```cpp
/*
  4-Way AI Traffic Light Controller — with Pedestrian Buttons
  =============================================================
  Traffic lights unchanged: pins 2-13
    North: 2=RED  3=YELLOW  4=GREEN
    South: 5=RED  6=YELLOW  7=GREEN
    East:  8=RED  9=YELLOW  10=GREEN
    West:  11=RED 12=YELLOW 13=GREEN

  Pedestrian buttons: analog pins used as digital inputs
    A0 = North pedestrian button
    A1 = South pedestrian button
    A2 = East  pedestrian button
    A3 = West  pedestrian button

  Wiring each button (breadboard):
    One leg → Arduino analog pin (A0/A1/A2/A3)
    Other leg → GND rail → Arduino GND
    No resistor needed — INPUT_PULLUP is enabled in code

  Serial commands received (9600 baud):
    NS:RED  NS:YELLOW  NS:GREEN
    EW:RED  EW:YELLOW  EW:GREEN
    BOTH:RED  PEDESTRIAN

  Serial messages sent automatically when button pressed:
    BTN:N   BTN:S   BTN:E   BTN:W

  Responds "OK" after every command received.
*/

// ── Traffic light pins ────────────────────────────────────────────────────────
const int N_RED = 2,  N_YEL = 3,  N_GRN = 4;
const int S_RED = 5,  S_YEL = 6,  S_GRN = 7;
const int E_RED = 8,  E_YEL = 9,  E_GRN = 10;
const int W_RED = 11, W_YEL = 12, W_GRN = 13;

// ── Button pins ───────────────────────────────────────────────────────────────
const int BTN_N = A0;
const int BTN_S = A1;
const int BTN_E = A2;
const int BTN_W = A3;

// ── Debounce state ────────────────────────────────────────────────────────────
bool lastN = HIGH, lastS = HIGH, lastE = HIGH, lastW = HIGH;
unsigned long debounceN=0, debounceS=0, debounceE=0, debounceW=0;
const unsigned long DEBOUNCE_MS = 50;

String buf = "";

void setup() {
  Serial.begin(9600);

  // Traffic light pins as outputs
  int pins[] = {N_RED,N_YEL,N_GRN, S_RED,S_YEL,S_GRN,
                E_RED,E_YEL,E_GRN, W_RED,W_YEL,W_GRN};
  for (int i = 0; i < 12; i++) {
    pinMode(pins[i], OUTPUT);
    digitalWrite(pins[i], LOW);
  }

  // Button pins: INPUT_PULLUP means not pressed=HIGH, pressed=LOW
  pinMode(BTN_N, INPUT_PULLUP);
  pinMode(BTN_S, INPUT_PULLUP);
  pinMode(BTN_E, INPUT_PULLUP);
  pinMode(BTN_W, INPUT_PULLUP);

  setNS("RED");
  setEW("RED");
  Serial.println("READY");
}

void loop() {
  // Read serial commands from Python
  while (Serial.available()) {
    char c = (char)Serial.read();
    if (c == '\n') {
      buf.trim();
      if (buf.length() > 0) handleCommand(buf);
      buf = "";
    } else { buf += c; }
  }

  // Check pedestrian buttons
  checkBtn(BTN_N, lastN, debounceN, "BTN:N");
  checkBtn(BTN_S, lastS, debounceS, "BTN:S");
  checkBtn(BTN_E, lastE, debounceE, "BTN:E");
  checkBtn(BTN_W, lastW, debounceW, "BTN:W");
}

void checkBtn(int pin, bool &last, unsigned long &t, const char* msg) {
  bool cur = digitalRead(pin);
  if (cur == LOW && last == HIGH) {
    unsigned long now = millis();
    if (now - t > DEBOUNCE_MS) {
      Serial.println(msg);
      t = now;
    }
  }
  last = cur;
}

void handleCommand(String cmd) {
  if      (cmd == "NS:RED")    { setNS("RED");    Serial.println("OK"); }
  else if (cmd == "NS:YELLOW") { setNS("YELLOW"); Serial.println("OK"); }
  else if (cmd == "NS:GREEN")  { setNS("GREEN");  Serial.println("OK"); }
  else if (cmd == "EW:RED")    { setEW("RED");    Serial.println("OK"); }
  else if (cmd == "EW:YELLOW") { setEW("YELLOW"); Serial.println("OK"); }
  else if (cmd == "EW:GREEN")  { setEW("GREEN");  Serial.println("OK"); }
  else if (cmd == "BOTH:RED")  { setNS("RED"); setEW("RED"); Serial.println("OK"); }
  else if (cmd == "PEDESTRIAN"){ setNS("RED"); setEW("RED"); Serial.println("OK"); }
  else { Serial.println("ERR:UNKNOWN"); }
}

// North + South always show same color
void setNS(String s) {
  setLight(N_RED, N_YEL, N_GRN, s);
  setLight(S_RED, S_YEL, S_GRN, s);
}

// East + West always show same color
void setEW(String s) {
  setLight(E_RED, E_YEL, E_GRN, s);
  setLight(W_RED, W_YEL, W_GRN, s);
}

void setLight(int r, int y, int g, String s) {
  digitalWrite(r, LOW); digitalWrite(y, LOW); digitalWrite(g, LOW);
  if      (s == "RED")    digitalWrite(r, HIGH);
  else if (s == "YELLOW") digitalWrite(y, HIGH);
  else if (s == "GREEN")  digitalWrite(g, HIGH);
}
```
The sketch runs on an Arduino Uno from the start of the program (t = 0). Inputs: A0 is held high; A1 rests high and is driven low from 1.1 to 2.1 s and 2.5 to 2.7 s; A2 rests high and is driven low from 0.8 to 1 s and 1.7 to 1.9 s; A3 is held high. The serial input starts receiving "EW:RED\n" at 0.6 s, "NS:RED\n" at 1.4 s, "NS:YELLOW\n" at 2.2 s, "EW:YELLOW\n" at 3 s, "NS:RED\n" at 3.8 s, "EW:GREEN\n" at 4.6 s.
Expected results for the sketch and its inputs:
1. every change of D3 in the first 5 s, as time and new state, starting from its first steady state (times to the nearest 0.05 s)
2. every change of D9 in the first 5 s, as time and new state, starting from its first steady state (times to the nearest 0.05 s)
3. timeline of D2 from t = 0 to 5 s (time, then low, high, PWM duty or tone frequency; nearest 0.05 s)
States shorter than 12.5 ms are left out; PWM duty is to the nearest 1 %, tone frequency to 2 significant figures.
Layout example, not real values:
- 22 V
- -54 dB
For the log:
- 0 s low; 2.2 s high; 3.8 s low
- 0 s low; 3 s high; 4.6 s low
- 0 s high; 2.2 s low; 3.8 s high
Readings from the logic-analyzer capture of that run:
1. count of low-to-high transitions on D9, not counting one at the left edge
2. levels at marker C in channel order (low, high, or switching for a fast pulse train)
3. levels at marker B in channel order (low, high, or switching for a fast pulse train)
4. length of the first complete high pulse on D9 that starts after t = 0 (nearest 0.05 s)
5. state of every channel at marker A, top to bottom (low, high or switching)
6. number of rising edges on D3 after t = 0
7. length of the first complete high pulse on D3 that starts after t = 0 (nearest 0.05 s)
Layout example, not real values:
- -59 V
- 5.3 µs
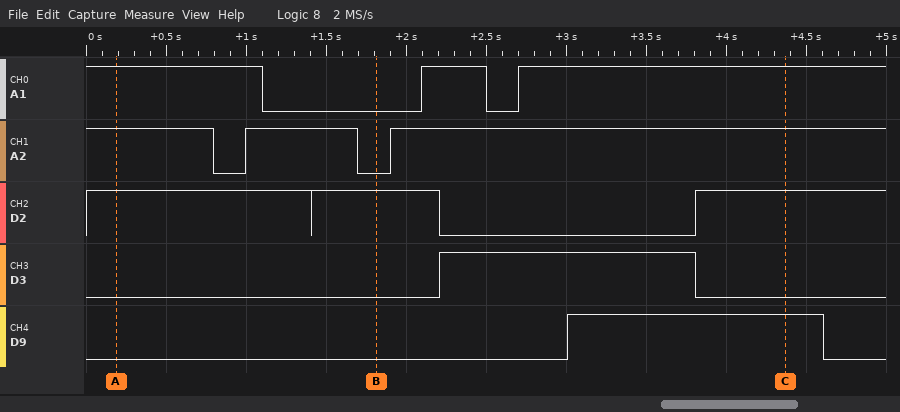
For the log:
- 1
- A1 high, A2 high, D2 high, D3 low, D9 high
- A1 low, A2 low, D2 high, D3 low, D9 low
- 1.60 s
- A1 high, A2 high, D2 high, D3 low, D9 low
- 1
- 1.60 s
